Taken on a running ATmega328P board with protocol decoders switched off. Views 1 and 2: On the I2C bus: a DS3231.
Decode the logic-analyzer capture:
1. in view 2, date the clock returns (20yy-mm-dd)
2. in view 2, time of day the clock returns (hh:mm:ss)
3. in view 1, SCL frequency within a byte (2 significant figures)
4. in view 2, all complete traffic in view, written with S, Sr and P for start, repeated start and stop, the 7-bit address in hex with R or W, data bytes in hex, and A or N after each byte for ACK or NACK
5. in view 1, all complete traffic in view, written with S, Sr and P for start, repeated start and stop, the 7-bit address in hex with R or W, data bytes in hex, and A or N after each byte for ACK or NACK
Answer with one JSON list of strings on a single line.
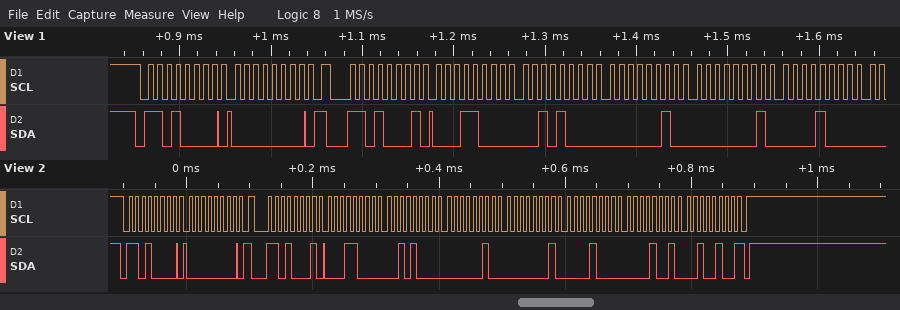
["2024-09-08", "02:28:18", "100 kHz", "S 68W A 00 A Sr 68R A 18 A 28 A 02 A 01 A 08 A 09 A 24 N P", "S 68W A 00 A Sr 68R A 18 A 28 A 02 A 01 A 08 A"]
